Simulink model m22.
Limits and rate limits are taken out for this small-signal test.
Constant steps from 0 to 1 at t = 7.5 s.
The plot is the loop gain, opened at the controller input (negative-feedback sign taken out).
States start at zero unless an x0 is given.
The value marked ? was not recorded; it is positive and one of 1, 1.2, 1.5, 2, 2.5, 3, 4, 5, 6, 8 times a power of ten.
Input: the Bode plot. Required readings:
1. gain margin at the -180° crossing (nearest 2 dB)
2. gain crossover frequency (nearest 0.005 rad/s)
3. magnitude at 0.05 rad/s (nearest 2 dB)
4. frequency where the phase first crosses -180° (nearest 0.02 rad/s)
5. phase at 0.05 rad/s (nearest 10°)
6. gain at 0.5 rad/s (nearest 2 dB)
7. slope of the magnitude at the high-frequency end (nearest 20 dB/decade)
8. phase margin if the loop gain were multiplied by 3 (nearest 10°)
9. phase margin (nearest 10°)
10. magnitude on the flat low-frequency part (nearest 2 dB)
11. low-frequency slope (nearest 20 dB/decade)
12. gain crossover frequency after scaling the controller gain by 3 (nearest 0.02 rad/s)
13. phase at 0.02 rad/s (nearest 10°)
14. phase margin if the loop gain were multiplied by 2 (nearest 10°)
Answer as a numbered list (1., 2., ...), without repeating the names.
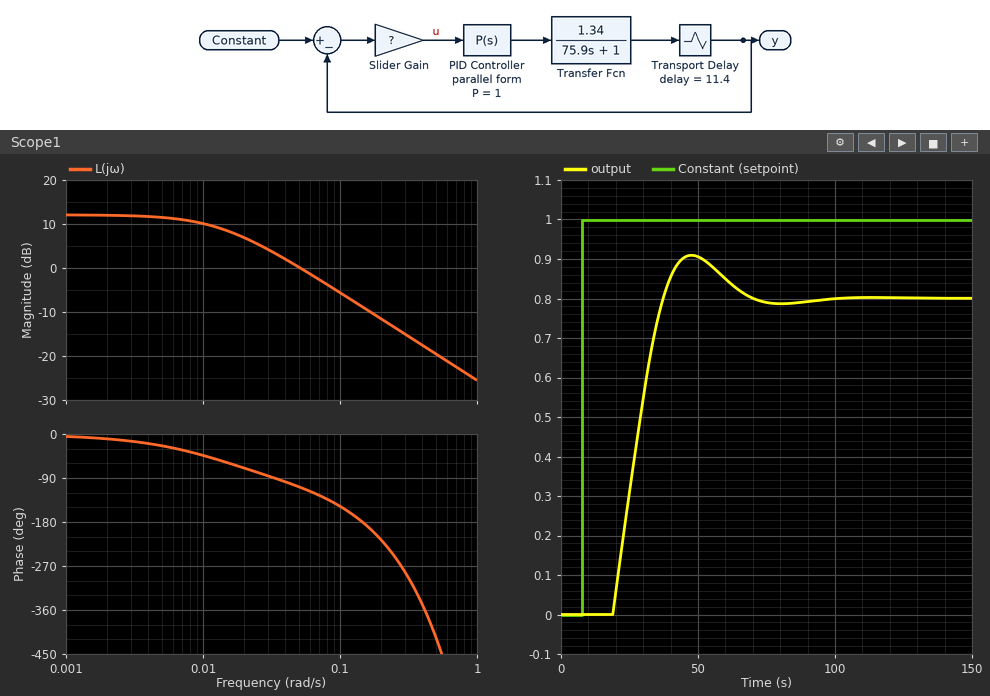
1. 8 dB
2. 0.050 rad/s
3. 0 dB
4. 0.14 rad/s
5. -110°
6. -20 dB
7. -20 dB/decade
8. -10°
9. 70°
10. 12 dB
11. 0 dB/decade
12. 0.16 rad/s
13. -70°
14. 30°
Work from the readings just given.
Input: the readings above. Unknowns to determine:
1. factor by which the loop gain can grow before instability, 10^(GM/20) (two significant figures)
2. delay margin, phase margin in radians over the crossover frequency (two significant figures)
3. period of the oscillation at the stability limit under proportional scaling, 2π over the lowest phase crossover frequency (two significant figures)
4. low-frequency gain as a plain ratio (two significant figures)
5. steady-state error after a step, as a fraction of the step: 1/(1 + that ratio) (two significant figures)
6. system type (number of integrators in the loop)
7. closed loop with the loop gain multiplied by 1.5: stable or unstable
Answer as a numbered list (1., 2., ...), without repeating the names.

1. 2.5
2. 24 s
3. 45 s
4. 4.0
5. 0.20
6. 0
7. stable
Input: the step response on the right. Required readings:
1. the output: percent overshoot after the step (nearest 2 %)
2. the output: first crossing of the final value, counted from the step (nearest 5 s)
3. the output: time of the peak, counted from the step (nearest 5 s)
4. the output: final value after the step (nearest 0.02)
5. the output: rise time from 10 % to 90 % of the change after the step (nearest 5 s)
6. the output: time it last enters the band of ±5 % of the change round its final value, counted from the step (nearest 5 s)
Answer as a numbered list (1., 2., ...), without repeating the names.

1. 14 %
2. 30 s
3. 40 s
4. 0.80
5. 15 s
6. 55 s
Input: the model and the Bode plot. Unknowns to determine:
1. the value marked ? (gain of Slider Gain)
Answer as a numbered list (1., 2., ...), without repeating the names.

1. 3
